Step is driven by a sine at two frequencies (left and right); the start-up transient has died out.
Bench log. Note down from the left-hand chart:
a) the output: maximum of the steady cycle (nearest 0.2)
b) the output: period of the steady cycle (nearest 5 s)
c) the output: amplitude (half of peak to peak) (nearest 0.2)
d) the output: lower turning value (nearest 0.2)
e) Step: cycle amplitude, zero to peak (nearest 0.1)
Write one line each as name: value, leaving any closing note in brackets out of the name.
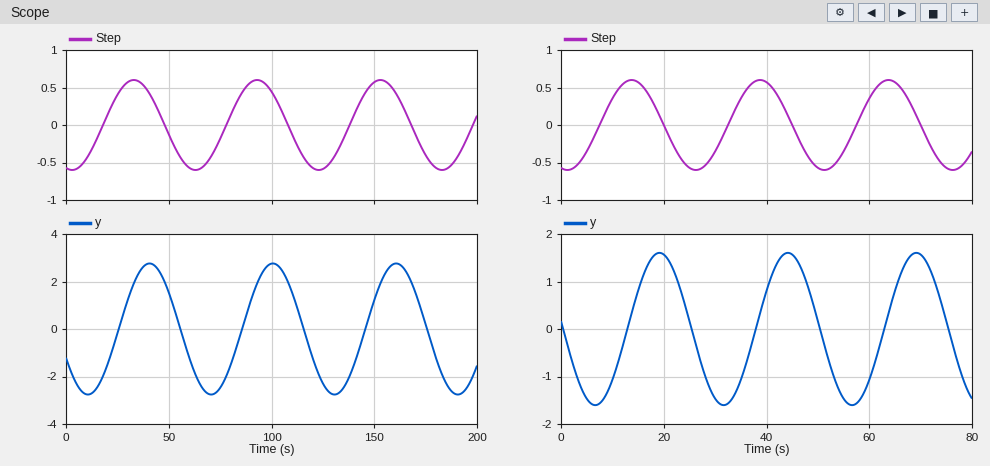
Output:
the output: maximum of the steady cycle: 2.8
the output: period of the steady cycle: 60 s
the output: amplitude (half of peak to peak): 2.8
the output: lower turning value: -2.8
Step: cycle amplitude, zero to peak: 0.6
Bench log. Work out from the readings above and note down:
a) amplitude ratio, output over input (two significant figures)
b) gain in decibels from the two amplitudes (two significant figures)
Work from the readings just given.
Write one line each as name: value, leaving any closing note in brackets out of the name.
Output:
amplitude ratio, output over input: 4.7
gain in decibels from the two amplitudes: 13 dB
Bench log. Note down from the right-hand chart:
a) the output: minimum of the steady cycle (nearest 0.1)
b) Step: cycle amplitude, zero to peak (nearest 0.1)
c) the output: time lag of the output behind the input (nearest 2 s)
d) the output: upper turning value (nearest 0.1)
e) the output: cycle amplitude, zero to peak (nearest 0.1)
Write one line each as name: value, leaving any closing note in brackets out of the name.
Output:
the output: minimum of the steady cycle: -1.6
Step: cycle amplitude, zero to peak: 0.6
the output: time lag of the output behind the input: 6 s
the output: upper turning value: 1.6
the output: cycle amplitude, zero to peak: 1.6
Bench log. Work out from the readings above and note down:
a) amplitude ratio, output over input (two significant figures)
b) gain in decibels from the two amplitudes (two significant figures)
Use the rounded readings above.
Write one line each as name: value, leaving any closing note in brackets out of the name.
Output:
amplitude ratio, output over input: 2.7
gain in decibels from the two amplitudes: 8.5 dB
